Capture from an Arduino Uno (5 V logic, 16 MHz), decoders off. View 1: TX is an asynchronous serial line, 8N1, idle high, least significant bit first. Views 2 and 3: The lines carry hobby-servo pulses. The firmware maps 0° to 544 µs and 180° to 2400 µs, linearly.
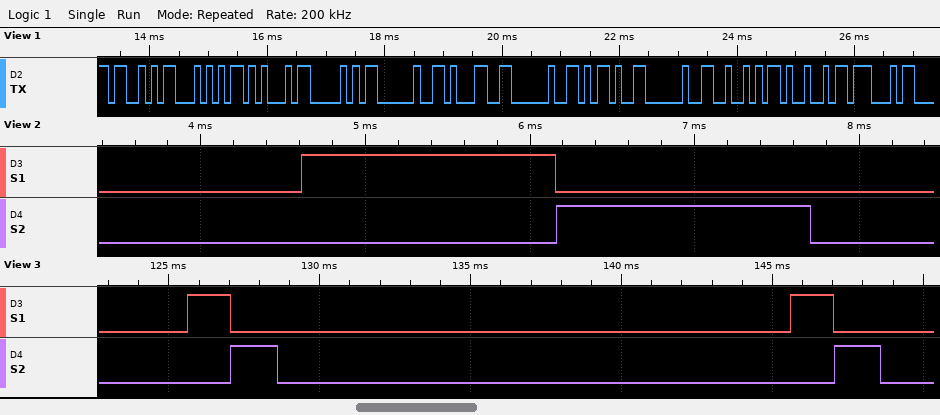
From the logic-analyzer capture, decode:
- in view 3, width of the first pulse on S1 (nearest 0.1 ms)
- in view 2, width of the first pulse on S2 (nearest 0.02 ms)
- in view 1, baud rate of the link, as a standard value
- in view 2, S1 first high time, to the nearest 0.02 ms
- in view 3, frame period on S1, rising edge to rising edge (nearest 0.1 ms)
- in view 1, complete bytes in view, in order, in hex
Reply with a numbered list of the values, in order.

1. 1.4 ms
2. 1.54 ms
3. 9600 baud
4. 1.54 ms
5. 20.0 ms
6. 53 54 45 50 20 31 20 2D 20 52 49 47
